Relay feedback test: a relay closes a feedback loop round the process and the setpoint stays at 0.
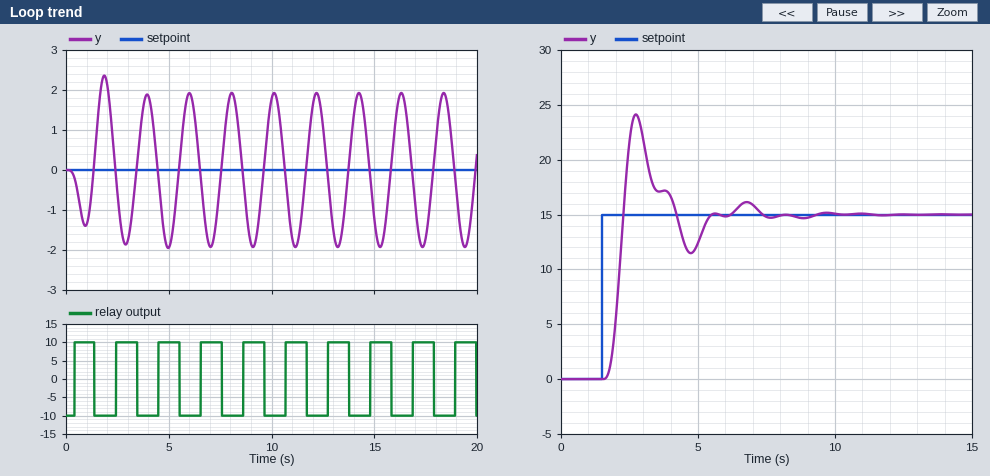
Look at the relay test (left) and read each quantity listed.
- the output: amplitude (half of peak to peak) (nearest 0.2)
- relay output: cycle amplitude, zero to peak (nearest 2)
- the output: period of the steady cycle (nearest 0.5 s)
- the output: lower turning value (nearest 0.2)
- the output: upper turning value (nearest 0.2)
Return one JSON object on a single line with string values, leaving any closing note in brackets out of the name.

{"the output: amplitude (half of peak to peak)": "2.0", "relay output: cycle amplitude, zero to peak": "10", "the output: period of the steady cycle": "2.0 s", "the output: lower turning value": "-2.0", "the output: upper turning value": "2.0"}
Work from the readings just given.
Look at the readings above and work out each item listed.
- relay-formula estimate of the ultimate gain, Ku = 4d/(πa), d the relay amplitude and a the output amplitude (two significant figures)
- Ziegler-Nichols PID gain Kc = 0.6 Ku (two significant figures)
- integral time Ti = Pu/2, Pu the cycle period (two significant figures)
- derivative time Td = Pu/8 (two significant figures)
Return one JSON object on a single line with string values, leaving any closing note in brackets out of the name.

{"relay-formula estimate of the ultimate gain, Ku = 4d/(πa), d the relay amplitude and a the output amplitude": "6.4", "Ziegler-Nichols PID gain Kc = 0.6 Ku": "3.8", "integral time Ti = Pu/2, Pu the cycle period": "1.0 s", "derivative time Td = Pu/8": "0.25 s"}
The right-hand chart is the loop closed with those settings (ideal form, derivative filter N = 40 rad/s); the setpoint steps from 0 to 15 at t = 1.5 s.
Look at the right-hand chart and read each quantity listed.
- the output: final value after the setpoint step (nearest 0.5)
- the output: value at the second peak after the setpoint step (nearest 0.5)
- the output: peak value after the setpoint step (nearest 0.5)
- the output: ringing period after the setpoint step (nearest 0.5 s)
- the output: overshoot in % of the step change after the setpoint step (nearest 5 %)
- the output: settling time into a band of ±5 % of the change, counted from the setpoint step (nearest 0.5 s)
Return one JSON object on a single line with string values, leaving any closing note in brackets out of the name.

{"the output: final value after the setpoint step": "15.0", "the output: value at the second peak after the setpoint step": "16.0", "the output: peak value after the setpoint step": "24.0", "the output: ringing period after the setpoint step": "4.0 s", "the output: overshoot in % of the step change after the setpoint step": "60 %", "the output: settling time into a band of ±5 % of the change, counted from the setpoint step": "5.5 s"}
